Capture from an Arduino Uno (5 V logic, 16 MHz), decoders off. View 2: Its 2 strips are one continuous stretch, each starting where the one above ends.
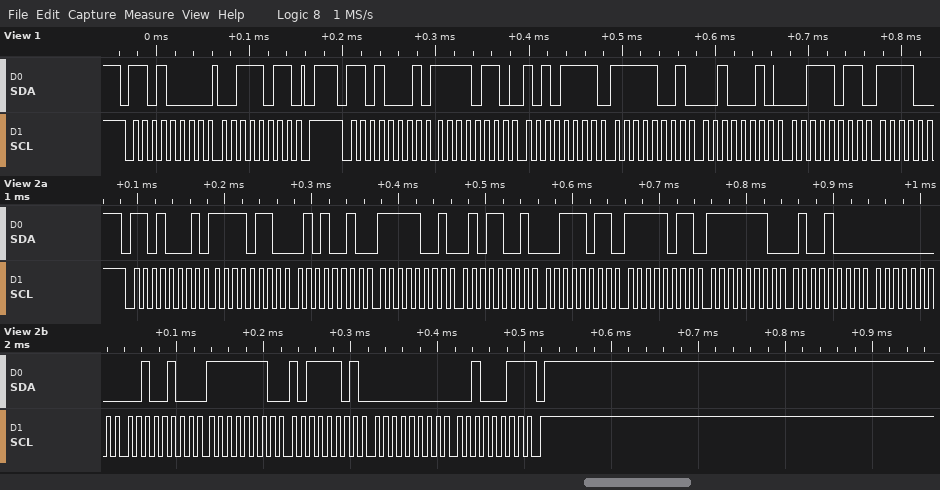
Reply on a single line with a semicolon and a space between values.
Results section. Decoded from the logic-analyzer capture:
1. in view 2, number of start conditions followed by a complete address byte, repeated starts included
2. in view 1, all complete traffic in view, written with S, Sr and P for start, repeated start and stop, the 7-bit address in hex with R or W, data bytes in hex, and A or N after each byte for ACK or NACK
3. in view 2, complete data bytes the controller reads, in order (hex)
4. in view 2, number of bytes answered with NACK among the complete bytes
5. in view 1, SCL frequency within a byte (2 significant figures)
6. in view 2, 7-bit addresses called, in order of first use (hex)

1; S 68W A 3B A P S 68R A F6 A AF A F9 A 22 A 3B A; F6 52 F9 59 3B FB FE 48 00 24 FE BD 00 23; 1; 100 kHz; 0x68
